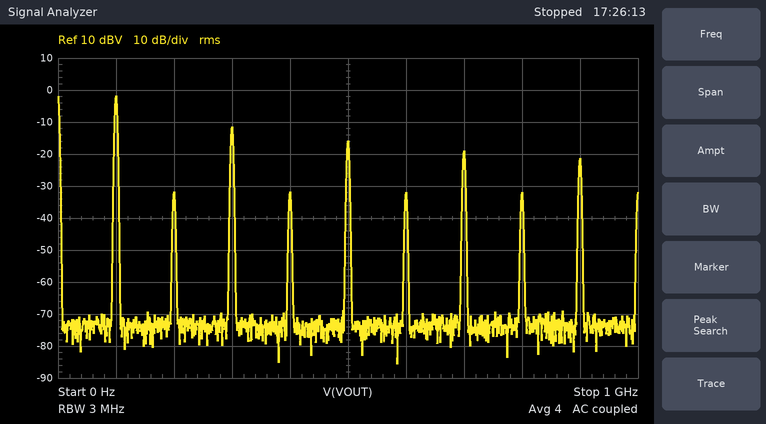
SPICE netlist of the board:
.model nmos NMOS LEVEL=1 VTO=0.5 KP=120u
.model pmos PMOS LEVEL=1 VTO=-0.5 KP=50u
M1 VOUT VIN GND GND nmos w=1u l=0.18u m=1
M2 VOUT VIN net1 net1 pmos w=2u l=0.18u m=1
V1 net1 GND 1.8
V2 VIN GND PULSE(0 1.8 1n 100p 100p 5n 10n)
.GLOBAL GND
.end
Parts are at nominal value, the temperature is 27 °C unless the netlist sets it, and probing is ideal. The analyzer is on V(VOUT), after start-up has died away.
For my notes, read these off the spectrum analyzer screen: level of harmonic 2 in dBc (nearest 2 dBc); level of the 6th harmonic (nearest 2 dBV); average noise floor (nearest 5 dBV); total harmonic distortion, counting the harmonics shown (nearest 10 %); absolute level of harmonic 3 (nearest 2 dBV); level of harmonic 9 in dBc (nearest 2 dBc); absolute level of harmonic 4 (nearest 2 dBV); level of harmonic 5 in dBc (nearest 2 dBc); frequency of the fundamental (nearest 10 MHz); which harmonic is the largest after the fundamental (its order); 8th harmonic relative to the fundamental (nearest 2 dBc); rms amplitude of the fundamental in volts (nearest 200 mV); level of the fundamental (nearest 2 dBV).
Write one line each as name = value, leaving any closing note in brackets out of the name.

level of harmonic 2 in dBc = -30 dBc
level of the 6th harmonic = -32 dBV
average noise floor = -75 dBV
total harmonic distortion, counting the harmonics shown = 40 %
absolute level of harmonic 3 = -12 dBV
level of harmonic 9 in dBc = -20 dBc
absolute level of harmonic 4 = -32 dBV
level of harmonic 5 in dBc = -14 dBc
frequency of the fundamental = 100 MHz
which harmonic is the largest after the fundamental = 3
8th harmonic relative to the fundamental = -30 dBc
rms amplitude of the fundamental in volts = 800 mV
level of the fundamental = -2 dBV
